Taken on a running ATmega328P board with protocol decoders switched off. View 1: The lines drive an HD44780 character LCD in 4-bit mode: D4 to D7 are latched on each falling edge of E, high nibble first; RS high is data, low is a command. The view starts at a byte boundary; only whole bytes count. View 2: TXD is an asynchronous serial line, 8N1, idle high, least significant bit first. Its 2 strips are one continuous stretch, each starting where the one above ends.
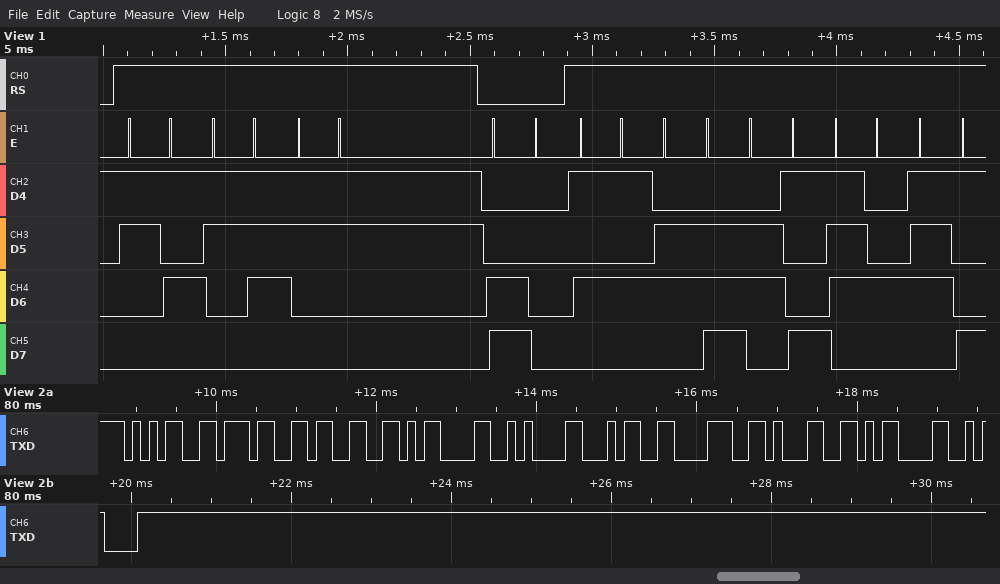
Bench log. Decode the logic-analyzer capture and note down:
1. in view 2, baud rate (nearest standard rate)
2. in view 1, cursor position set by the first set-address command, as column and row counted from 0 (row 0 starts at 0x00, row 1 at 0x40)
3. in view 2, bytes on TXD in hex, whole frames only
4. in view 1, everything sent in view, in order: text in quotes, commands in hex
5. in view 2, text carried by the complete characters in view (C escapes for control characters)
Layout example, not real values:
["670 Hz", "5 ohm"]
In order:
["9600 baud", "column 0, row 1", "35 37 33 0D 0A 34 38 31 0D 0A", "\"573\" 0xC0 \"Unity\"", "\"573\\r\\n481\\r\\n\""]
